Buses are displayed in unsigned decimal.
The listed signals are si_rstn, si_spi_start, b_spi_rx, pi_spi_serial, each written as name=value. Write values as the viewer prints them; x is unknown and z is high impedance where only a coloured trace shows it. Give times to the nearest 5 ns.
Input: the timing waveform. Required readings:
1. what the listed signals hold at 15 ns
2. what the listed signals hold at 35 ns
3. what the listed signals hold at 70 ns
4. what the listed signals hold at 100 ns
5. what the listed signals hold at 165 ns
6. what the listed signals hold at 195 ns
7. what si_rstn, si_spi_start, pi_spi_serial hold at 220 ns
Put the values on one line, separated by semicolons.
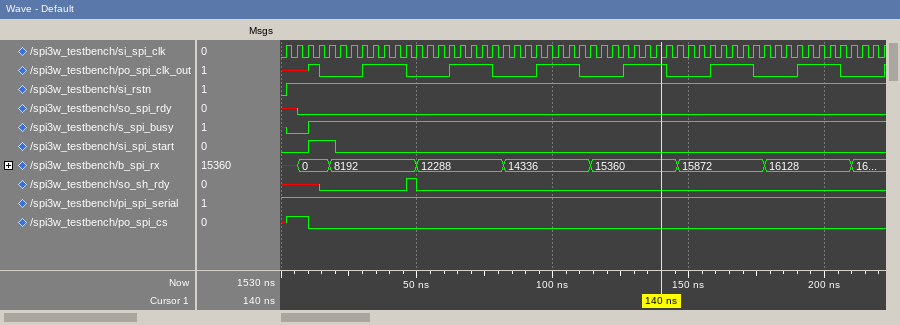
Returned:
si_rstn=1, si_spi_start=1, b_spi_rx=0, pi_spi_serial=1; si_rstn=1, si_spi_start=0, b_spi_rx=8192, pi_spi_serial=1; si_rstn=1, si_spi_start=0, b_spi_rx=12288, pi_spi_serial=1; si_rstn=1, si_spi_start=0, b_spi_rx=14336, pi_spi_serial=1; si_rstn=1, si_spi_start=0, b_spi_rx=15872, pi_spi_serial=1; si_rstn=1, si_spi_start=0, b_spi_rx=16128, pi_spi_serial=1; si_rstn=1, si_spi_start=0, pi_spi_serial=1
